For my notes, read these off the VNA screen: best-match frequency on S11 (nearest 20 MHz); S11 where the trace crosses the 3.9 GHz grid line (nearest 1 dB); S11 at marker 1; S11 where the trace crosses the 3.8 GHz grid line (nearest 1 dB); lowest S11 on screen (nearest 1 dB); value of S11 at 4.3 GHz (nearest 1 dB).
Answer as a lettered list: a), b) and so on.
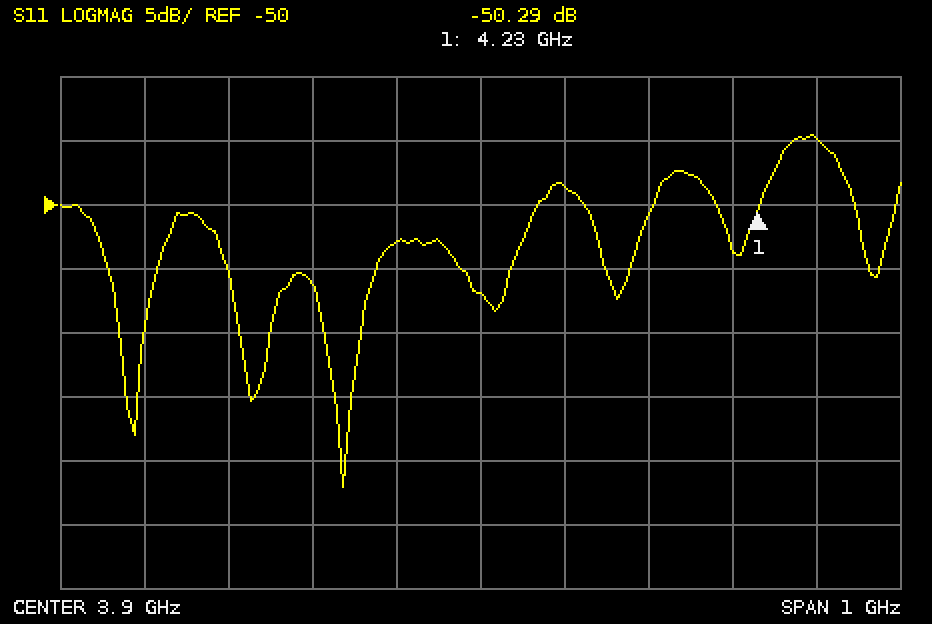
a) 3.74 GHz
b) -57 dB
c) -50.29 dB
d) -53 dB
e) -72 dB
f) -45 dB
